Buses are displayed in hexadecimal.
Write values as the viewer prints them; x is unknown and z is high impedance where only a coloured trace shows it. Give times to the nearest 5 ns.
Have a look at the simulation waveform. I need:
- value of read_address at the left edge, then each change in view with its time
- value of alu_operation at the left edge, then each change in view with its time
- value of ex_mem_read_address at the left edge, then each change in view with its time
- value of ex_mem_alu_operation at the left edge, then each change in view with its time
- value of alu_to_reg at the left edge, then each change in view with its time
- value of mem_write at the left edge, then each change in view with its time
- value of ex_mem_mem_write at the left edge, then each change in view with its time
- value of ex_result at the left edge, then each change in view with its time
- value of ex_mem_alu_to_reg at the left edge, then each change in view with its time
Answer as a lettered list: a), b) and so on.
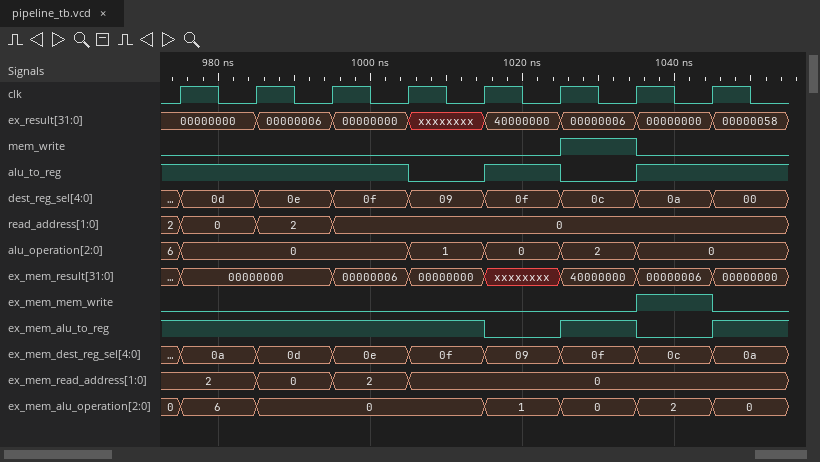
a) 2, 0 at 975 ns, 2 at 985 ns, 0 at 995 ns
b) 6, 0 at 975 ns, 1 at 1005 ns, 0 at 1015 ns, 2 at 1025 ns, 0 at 1035 ns
c) 2, 0 at 985 ns, 2 at 995 ns, 0 at 1005 ns
d) 0, 6 at 975 ns, 0 at 985 ns, 1 at 1015 ns, 0 at 1025 ns, 2 at 1035 ns, 0 at 1045 ns
e) 1, 0 at 1005 ns, 1 at 1015 ns, 0 at 1025 ns, 1 at 1035 ns
f) 0, 1 at 1025 ns, 0 at 1035 ns
g) 0, 1 at 1035 ns, 0 at 1045 ns
h) 00000000, 00000006 at 985 ns, 00000000 at 995 ns, xxxxxxxx at 1005 ns, 40000000 at 1015 ns, 00000006 at 1025 ns, 00000000 at 1035 ns, 00000058 at 1045 ns
i) 1, 0 at 1015 ns, 1 at 1025 ns, 0 at 1035 ns, 1 at 1045 ns
